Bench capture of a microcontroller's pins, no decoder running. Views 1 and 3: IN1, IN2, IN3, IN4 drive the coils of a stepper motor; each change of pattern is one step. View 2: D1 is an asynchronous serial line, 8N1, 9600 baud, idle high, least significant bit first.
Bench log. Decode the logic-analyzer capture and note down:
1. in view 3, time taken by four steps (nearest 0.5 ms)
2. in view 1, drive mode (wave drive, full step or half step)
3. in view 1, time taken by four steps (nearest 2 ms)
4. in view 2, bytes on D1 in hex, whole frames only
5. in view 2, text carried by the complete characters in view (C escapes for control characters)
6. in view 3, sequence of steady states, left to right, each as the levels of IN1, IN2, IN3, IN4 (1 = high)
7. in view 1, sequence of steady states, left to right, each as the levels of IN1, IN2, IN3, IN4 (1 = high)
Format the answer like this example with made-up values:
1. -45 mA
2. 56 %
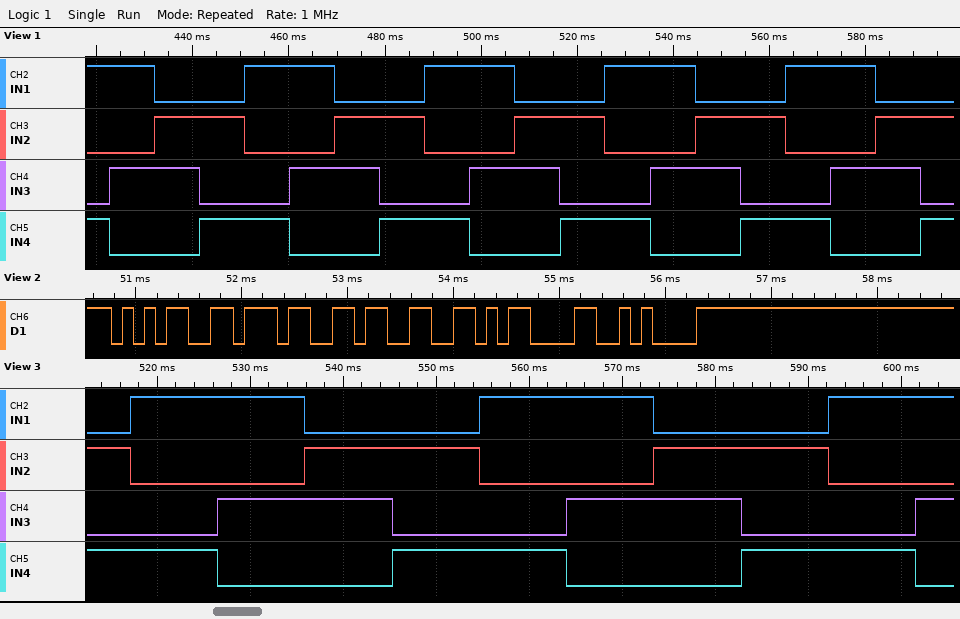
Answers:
1. 37.5 ms
2. full step
3. 38 ms
4. 35 37 33 0D 0A
5. "573\r\n"
6. 0101 1001 1010 0110 0101 1001 1010 0110 0101 1001 1010
7. 1001 1010 0110 0101 1001 1010 0110 0101 1001 1010 0110 0101 1001 1010 0110 0101 1001 1010 0110 0101
